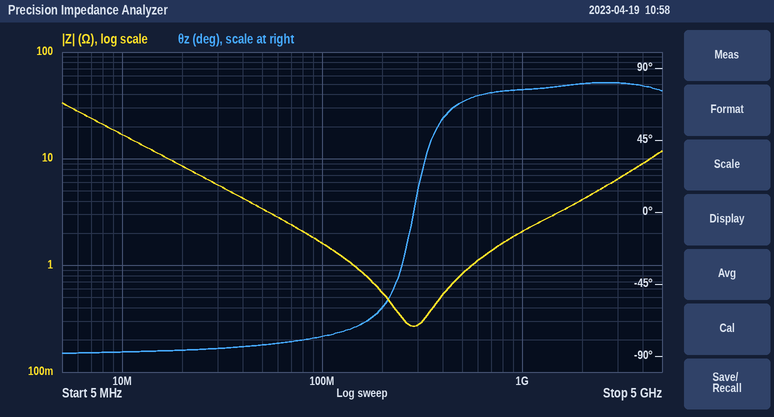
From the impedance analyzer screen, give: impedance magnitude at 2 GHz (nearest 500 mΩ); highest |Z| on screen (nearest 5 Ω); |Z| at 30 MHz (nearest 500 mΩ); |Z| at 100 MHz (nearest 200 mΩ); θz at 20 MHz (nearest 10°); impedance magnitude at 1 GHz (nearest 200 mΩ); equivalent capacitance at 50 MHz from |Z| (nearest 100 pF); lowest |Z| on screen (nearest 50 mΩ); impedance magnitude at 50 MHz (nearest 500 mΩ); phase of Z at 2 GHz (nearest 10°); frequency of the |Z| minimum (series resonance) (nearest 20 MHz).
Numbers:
4.0 Ω
35 Ω
5.5 Ω
1.6 Ω
-90°
2.0 Ω
900 pF
250 mΩ
3.5 Ω
80°
280 MHz
